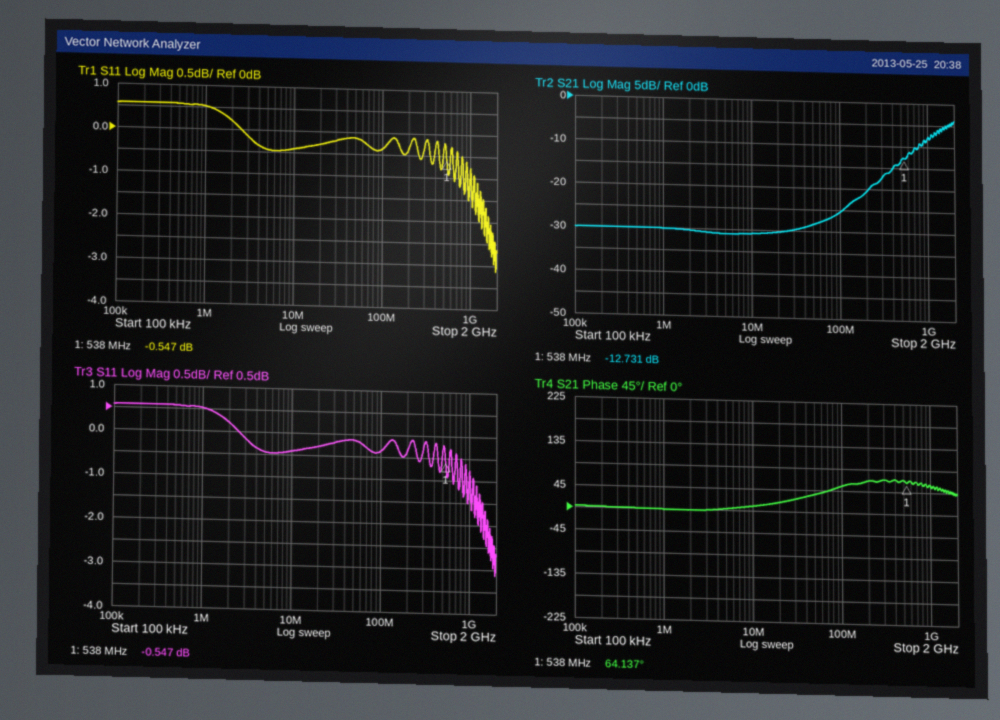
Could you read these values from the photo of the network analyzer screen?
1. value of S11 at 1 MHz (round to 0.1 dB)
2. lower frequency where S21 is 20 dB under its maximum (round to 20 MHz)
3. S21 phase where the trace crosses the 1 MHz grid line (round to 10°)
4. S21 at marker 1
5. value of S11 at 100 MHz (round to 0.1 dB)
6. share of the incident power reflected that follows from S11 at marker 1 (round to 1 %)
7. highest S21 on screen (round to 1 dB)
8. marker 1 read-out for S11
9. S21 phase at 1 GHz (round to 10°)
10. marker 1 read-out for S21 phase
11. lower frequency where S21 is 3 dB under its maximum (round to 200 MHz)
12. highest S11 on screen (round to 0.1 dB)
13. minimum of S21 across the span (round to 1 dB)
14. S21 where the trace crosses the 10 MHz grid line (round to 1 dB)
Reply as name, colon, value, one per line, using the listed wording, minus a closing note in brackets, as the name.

value of S11 at 1 MHz: 0.5 dB
lower frequency where S21 is 20 dB under its maximum: 120 MHz
S21 phase where the trace crosses the 1 MHz grid line: 0°
S21 at marker 1: -12.731 dB
value of S11 at 100 MHz: -0.4 dB
share of the incident power reflected that follows from S11 at marker 1: 88 %
highest S21 on screen: -4 dB
marker 1 read-out for S11: -0.547 dB
S21 phase at 1 GHz: 60°
marker 1 read-out for S21 phase: 64.137°
lower frequency where S21 is 3 dB under its maximum: 1.2 GHz
highest S11 on screen: 0.6 dB
minimum of S21 across the span: -31 dB
S21 where the trace crosses the 10 MHz grid line: -31 dB
